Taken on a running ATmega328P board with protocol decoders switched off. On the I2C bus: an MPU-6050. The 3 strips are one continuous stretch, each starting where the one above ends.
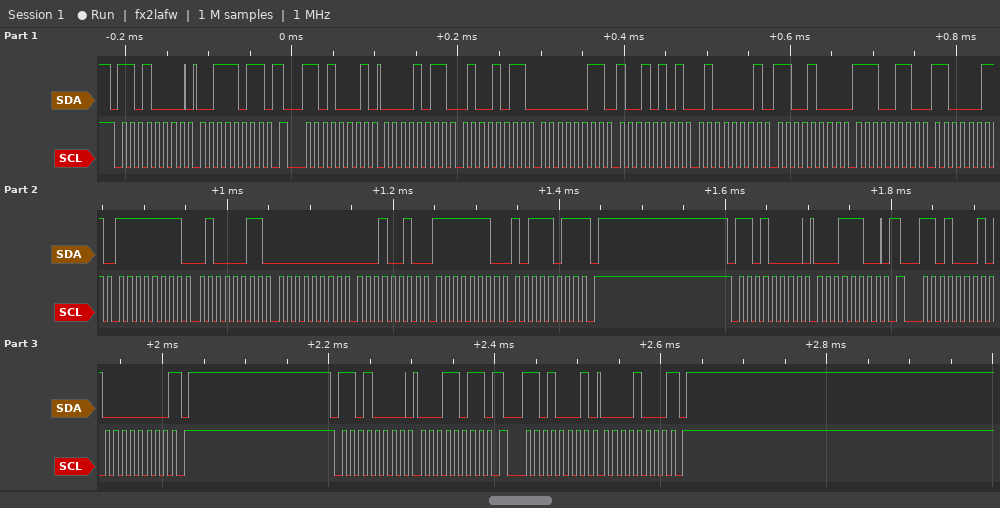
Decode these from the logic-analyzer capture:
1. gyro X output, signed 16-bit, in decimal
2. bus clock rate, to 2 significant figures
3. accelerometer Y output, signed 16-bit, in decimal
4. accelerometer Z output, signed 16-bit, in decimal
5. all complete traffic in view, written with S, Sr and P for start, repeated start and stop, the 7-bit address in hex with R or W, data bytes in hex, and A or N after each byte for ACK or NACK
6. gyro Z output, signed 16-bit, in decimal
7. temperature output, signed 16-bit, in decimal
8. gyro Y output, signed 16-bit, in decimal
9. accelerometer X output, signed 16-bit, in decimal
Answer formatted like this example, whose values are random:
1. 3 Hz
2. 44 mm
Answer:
1. -189
2. 100 kHz
3. 917
4. 16840
5. S 68W A 3B A Sr 68R A 0B A 4B A 03 A 95 A 41 A C8 A E6 A C3 A FF A 43 A 00 A 12 A FE A BB N P S 68W A 1C A Sr 68R A 00 N P S 68W A 1B A Sr 68R A 08 N P
6. -325
7. -6461
8. 18
9. 2891
